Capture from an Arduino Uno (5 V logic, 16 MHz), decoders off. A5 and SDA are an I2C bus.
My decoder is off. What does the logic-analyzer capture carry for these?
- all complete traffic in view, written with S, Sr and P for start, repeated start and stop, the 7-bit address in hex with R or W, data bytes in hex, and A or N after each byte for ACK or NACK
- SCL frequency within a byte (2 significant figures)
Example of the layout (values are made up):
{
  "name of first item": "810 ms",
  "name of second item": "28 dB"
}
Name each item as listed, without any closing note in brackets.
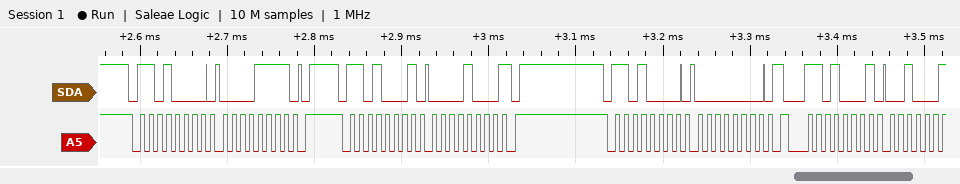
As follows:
{
  "all complete traffic in view, written with S, Sr and P for start, repeated start and stop, the 7-bit address in hex with R or W, data bytes in hex, and A or N after each byte for ACK or NACK": "S 68W A 0F A P S 68R A 08 N P S 68W A 00 A Sr 68R A",
  "SCL frequency within a byte": "100 kHz"
}
